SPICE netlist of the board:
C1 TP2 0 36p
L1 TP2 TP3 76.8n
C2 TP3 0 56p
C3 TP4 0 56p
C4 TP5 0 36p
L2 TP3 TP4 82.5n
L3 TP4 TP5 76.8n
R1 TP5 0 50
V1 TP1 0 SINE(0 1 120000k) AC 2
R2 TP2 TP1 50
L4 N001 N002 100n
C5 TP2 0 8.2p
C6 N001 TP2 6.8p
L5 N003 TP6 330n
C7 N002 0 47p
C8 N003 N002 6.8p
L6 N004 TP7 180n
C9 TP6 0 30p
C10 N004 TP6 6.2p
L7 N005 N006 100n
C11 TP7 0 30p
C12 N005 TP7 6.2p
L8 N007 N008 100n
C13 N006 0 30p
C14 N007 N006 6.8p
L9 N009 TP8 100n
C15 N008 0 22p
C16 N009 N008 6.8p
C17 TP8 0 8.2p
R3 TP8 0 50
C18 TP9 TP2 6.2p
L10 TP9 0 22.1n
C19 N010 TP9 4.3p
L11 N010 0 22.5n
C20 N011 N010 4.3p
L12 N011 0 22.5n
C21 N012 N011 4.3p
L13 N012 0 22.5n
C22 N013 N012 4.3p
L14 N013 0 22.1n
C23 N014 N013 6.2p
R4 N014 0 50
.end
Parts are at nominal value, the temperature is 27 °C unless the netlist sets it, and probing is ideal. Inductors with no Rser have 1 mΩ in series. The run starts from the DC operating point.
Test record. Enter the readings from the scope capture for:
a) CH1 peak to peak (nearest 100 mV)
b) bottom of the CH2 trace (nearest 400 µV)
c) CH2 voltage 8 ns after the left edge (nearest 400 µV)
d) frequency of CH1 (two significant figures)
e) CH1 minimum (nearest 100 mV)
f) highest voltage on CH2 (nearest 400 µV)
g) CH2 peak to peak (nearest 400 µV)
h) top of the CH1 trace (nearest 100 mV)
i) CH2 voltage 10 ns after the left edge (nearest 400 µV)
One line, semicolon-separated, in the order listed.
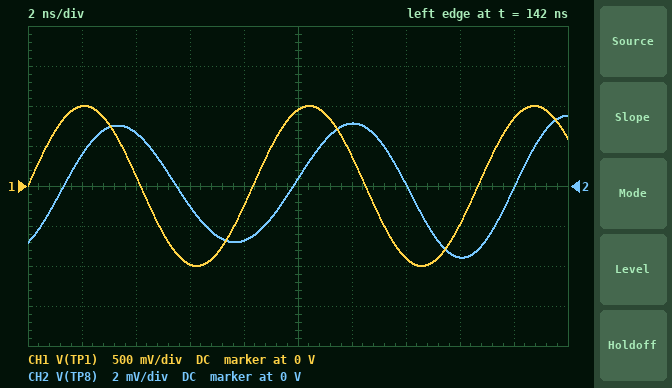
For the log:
2.0 V; -3.6 mV; -2.8 mV; 120 MHz; -1.0 V; 3.6 mV; 7.2 mV; 1.0 V; 400 µV
